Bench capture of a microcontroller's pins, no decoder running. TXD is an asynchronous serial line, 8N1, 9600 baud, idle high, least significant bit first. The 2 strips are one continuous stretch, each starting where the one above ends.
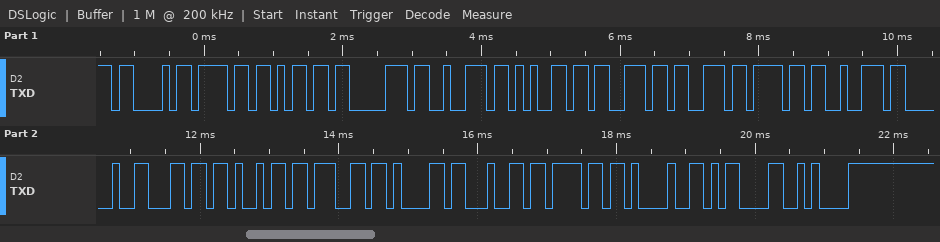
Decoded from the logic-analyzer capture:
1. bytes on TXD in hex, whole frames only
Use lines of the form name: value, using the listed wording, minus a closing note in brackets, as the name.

bytes on TXD in hex, whole frames only: 0x43 0x6F 0x6D 0x70 0x72 0x65 0x73 0x73 0x6F 0x72 0x20 0x6C 0x69 0x67 0x61 0x64 0x6F 0x21 0x0D 0x0A
